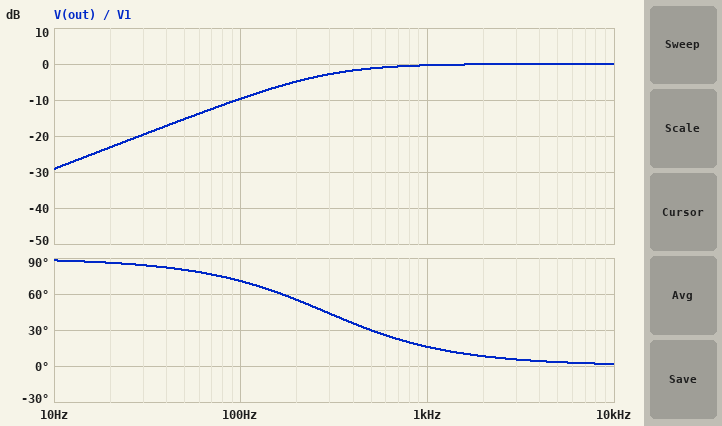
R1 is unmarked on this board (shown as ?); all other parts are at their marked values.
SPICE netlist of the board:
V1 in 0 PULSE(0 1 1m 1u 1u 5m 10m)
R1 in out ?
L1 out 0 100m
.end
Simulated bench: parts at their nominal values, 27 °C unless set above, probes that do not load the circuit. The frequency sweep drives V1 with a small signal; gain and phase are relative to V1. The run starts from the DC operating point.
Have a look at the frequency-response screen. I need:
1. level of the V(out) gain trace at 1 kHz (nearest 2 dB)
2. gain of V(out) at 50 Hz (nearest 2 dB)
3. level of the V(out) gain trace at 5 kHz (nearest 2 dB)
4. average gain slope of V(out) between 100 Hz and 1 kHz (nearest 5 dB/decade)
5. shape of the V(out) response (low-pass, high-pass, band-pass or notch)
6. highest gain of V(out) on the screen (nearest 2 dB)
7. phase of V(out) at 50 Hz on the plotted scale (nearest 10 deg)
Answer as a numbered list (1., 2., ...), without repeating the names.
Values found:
1. 0 dB
2. -16 dB
3. 0 dB
4. 10 dB/decade
5. high-pass
6. 0 dB
7. 80 deg
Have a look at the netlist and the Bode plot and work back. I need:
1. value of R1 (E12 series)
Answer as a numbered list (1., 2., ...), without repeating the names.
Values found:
1. 180 Ω
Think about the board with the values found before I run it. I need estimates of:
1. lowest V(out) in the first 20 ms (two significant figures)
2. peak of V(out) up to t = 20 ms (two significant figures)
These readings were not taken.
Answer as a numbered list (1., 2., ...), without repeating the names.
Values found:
1. -1.0 V
2. 1.0 V
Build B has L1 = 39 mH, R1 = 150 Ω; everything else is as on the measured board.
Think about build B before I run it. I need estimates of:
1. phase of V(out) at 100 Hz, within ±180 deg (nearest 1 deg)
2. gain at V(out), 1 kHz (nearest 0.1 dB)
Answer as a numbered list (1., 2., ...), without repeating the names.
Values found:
1. 81 deg
2. -1.4 dB
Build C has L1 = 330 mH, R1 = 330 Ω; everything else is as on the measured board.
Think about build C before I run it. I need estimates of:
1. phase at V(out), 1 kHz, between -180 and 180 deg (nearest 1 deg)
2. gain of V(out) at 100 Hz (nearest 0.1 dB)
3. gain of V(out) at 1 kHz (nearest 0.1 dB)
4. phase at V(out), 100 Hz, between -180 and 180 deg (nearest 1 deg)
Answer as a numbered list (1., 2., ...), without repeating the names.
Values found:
1. 9 deg
2. -5.5 dB
3. -0.1 dB
4. 58 deg
